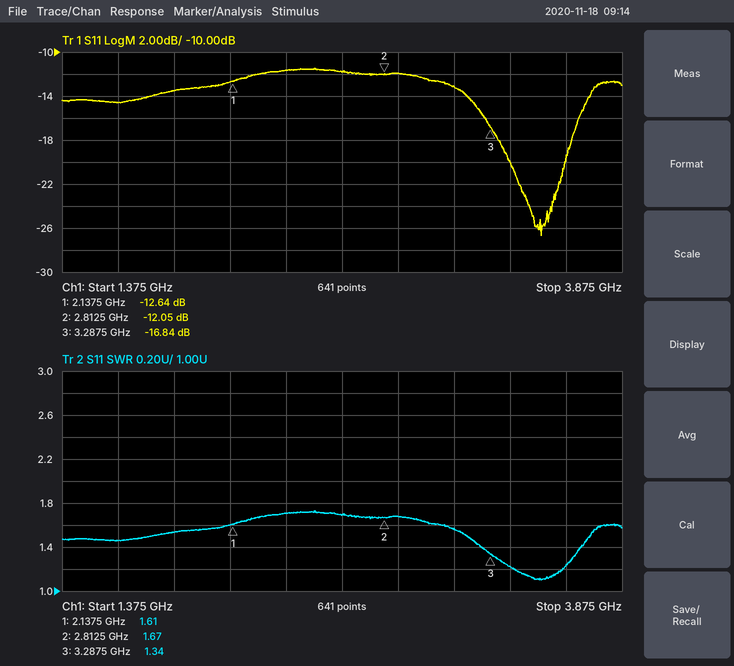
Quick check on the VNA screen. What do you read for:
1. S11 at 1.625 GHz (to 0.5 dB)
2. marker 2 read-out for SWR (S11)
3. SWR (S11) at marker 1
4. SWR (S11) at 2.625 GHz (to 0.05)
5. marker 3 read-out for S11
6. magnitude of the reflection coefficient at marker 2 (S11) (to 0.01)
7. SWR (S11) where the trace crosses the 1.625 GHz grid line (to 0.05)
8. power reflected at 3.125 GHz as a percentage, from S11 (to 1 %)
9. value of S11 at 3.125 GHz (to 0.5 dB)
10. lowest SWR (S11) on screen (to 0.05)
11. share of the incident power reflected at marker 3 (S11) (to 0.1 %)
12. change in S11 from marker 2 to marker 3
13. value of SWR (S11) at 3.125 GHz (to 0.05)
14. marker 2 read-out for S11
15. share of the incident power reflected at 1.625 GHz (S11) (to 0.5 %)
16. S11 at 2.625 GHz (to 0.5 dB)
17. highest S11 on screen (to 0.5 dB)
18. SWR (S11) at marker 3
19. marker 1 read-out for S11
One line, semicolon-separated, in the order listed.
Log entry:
-14.5 dB; 1.67; 1.61; 1.70; -16.84 dB; 0.25; 1.45; 5 %; -13.0 dB; 1.10; 2.1 %; -4.79 dB; 1.55; -12.05 dB; 3.5 %; -12.0 dB; -11.5 dB; 1.34; -12.64 dB
